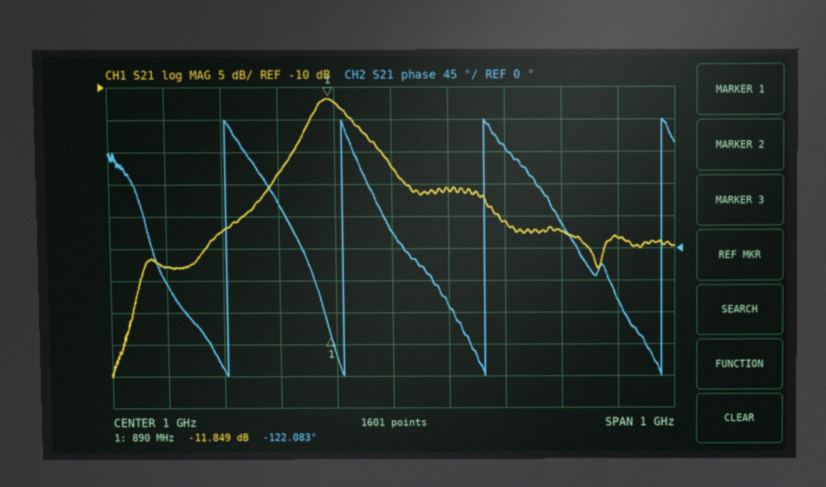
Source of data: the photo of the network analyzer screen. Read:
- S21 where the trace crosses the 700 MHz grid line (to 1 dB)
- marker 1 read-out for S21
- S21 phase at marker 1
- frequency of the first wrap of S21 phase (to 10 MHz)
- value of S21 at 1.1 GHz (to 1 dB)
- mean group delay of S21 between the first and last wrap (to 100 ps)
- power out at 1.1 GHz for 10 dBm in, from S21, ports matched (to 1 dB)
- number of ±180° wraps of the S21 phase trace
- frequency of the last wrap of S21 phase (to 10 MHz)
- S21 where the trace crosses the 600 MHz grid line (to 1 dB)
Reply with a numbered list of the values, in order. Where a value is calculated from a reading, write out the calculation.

1. -32 dB
2. -11.849 dB
3. -122.083°
4. 710 MHz
5. -26 dB
6. 3 cycles / (1.48 GHz − 710 MHz) ≈ 3.9 ns
7. 10 dBm + (-26 dB) = -16 dBm
8. 4
9. 1.48 GHz
10. -38 dB
